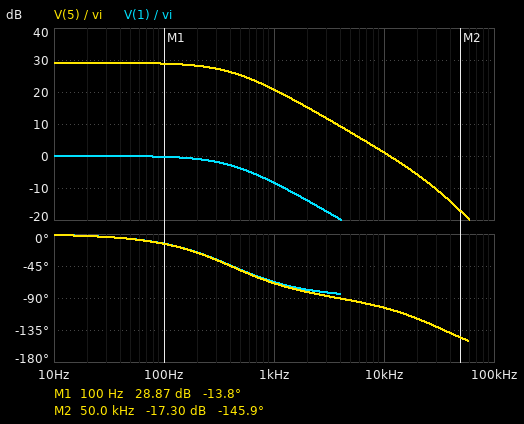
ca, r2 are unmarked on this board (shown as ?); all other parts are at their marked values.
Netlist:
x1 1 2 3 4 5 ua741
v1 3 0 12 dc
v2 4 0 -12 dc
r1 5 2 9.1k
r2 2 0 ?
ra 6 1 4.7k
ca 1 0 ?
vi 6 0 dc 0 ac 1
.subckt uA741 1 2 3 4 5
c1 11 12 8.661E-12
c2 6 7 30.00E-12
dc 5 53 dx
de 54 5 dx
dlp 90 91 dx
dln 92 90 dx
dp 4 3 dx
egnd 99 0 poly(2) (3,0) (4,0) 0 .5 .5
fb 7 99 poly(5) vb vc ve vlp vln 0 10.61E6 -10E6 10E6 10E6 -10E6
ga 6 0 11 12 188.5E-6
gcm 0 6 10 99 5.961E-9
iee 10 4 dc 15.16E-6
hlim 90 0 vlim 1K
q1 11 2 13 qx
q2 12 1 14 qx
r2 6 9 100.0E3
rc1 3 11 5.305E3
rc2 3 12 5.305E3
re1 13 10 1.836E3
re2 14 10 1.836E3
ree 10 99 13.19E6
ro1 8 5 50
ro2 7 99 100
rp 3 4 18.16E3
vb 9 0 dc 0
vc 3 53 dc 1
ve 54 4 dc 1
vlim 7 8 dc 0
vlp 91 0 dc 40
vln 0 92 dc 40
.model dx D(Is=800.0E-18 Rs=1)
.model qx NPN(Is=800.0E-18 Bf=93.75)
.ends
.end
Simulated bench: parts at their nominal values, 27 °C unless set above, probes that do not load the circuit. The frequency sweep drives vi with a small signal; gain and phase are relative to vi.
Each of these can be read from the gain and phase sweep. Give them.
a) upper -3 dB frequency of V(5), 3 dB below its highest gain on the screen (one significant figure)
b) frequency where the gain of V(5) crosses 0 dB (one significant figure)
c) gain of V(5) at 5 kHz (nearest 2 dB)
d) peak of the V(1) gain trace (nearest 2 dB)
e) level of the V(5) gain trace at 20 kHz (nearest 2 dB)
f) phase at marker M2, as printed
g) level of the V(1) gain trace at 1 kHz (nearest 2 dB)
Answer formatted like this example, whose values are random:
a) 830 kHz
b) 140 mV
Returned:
a) 400 Hz
b) 10 kHz
c) 8 dB
d) 0 dB
e) -6 dB
f) -145.9 deg
g) -8 dB
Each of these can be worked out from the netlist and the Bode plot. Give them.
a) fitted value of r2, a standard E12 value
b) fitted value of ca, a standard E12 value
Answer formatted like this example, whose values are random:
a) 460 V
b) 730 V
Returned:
a) 330 Ω
b) 82 nF
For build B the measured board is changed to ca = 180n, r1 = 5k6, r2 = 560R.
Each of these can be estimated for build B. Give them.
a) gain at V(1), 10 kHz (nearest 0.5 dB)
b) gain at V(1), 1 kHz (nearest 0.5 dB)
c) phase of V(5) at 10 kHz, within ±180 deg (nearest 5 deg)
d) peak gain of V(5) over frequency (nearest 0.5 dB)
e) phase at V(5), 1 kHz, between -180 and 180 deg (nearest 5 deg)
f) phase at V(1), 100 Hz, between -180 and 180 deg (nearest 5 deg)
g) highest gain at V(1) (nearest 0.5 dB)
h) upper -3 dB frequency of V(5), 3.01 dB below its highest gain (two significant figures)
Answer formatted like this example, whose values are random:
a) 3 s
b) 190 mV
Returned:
a) -34.5 dB
b) -14.5 dB
c) -95 deg
d) 21.0 dB
e) -80 deg
f) -30 deg
g) 0 dB
h) 190 Hz
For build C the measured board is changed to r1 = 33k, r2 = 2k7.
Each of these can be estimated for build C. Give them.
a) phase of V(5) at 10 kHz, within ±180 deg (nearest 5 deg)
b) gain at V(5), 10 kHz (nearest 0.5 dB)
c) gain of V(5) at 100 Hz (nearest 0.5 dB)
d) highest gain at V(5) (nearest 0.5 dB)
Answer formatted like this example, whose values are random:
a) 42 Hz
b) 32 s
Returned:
a) -95 deg
b) -5.5 dB
c) 22.0 dB
d) 22.5 dB
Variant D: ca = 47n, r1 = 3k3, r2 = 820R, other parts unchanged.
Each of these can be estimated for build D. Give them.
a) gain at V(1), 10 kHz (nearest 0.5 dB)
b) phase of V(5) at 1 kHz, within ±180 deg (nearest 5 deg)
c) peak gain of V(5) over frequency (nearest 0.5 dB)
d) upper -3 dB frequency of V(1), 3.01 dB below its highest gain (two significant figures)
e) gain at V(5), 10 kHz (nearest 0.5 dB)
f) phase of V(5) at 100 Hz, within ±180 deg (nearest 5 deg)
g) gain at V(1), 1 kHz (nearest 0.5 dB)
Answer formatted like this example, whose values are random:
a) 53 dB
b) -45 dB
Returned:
a) -23.0 dB
b) -55 deg
c) 14.0 dB
d) 720 Hz
e) -9.0 dB
f) -10 deg
g) -4.5 dB
